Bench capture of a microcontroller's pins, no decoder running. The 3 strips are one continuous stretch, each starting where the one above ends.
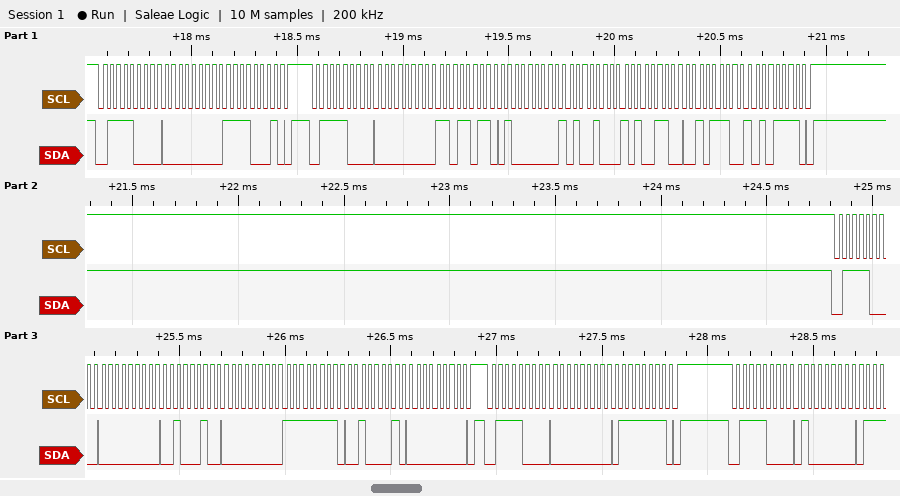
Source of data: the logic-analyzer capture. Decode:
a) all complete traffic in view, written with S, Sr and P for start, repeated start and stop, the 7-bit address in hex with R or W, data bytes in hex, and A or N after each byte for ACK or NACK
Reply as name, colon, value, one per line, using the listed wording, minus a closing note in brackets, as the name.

all complete traffic in view, written with S, Sr and P for start, repeated start and stop, the 7-bit address in hex with R or W, data bytes in hex, and A or N after each byte for ACK or NACK: S 3CW A 00 A F1 A P S 3CW A 00 A DB A 40 A A4 A A6 A 2E A AF A P S 3CW A 00 A 22 A 00 A FF A 21 A 00 A P S 3CW A 00 A 7F A P S 3CW A 40 A
